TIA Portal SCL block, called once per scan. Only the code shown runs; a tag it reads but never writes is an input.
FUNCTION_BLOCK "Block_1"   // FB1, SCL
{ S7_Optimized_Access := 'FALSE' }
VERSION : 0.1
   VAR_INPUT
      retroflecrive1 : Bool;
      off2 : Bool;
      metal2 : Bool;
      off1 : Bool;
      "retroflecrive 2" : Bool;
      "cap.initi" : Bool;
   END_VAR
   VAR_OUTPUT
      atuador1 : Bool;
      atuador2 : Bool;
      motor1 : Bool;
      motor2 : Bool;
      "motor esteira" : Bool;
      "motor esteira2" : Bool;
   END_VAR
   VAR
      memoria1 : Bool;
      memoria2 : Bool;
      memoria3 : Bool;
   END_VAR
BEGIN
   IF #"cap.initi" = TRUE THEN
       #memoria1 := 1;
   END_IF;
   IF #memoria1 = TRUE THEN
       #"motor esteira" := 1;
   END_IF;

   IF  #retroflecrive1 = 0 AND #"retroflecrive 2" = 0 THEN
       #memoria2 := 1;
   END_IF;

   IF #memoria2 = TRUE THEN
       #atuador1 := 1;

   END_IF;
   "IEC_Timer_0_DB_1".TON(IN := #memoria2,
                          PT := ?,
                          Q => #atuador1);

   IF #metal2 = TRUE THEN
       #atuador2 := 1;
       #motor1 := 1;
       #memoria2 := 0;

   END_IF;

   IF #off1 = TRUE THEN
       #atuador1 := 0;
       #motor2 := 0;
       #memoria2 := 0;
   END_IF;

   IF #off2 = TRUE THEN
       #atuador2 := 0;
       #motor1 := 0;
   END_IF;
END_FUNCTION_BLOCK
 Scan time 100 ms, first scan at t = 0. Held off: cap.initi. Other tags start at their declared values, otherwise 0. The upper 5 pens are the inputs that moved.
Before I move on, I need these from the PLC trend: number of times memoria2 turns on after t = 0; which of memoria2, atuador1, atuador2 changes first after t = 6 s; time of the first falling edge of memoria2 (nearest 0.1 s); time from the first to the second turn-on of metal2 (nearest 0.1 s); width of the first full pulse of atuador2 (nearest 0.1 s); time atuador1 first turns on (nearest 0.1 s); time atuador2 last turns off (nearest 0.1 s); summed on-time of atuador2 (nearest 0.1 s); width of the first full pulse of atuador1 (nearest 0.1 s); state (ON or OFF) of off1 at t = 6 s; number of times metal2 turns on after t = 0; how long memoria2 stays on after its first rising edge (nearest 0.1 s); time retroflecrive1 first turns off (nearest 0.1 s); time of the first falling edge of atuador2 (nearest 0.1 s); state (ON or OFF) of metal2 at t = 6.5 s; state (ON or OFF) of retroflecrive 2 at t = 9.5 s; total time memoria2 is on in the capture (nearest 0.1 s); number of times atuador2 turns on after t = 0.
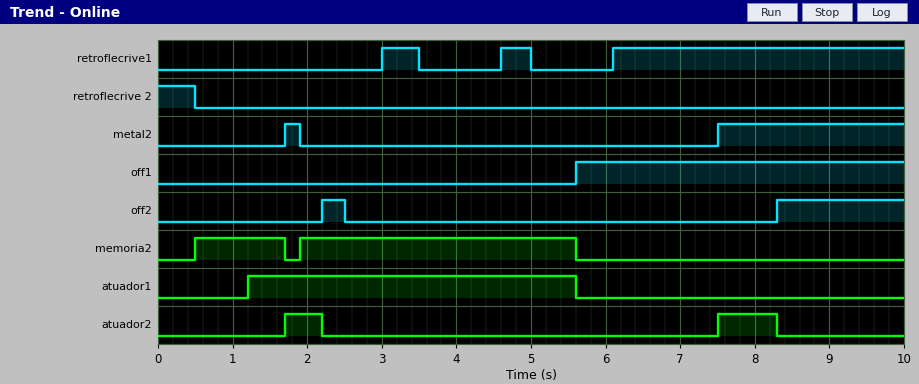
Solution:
2
atuador2
1.7 s
5.8 s
0.5 s
1.2 s
8.3 s
1.3 s
4.4 s
ON
2
1.2 s
3.5 s
2.2 s
OFF
OFF
4.9 s
2
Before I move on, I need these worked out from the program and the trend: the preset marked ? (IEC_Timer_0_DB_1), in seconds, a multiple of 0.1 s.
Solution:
0.7 s
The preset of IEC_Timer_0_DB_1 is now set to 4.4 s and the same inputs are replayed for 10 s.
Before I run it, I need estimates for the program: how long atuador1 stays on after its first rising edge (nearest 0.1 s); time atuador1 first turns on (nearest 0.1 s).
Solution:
0.7 s
4.9 s
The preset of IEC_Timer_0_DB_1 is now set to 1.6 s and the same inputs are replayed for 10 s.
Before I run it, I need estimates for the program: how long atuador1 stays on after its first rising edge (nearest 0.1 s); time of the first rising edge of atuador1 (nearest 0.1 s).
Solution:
3.5 s
2.1 s
